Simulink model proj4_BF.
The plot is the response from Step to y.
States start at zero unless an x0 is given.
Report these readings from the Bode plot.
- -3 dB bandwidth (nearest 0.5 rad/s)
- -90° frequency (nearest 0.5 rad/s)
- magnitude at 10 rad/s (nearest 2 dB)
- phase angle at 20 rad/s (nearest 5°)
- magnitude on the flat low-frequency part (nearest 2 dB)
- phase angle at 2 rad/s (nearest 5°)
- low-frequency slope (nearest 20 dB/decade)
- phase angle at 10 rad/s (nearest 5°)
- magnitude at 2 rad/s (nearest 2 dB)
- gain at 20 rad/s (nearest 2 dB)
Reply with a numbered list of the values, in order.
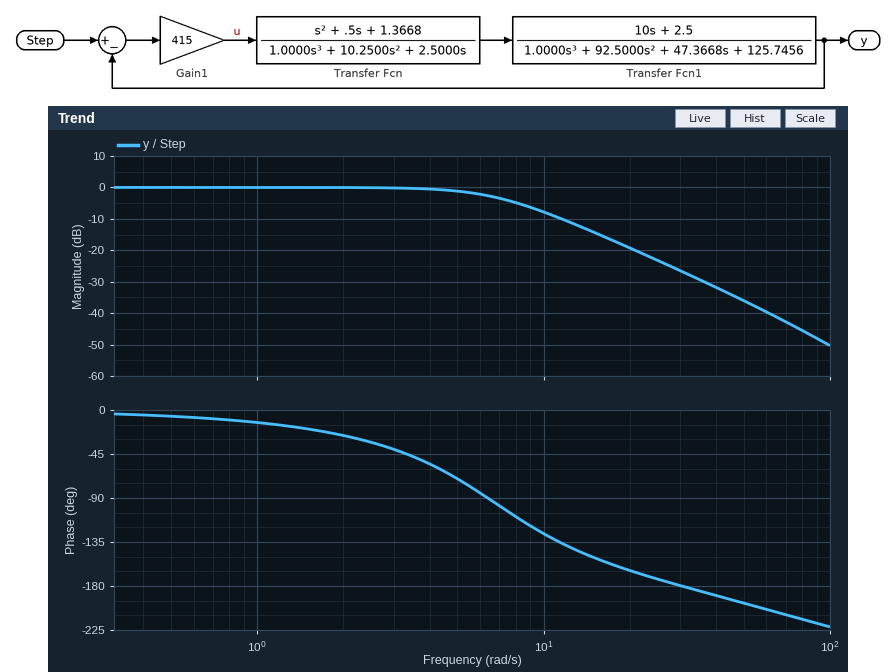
1. 6.5 rad/s
2. 6.5 rad/s
3. -8 dB
4. -165°
5. 0 dB
6. -25°
7. 0 dB/decade
8. -125°
9. 0 dB
10. -20 dB
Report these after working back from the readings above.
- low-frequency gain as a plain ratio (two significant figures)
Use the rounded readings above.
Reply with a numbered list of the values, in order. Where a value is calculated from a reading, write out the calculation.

1. 10^(0 / 20) = 1.0
